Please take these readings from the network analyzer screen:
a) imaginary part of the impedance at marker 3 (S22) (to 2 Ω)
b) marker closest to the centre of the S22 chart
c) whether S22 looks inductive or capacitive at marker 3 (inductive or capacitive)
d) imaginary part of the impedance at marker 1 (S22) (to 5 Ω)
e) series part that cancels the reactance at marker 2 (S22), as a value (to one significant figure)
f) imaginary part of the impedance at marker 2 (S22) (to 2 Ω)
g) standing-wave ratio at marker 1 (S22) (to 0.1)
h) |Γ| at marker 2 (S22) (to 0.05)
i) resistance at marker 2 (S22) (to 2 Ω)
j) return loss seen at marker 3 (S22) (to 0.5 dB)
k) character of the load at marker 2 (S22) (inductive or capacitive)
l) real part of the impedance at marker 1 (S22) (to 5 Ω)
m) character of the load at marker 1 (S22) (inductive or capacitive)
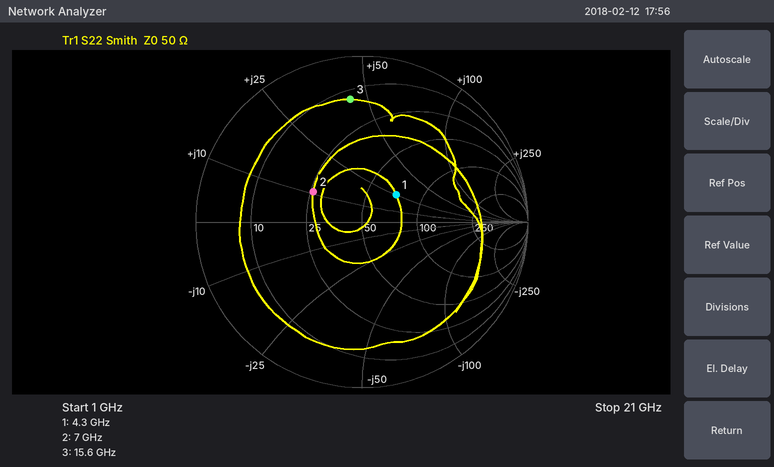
+44 Ω
marker 1
inductive
+25 Ω
2 pF
+10 Ω
1.7
0.35
26 Ω
2.5 dB
inductive
70 Ω
inductive
